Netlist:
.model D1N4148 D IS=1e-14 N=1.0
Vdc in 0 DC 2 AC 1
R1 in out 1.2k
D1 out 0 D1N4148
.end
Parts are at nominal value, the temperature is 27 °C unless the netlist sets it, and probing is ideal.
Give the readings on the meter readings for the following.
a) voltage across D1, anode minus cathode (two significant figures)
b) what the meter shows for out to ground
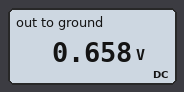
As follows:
660 mV
0.658 V
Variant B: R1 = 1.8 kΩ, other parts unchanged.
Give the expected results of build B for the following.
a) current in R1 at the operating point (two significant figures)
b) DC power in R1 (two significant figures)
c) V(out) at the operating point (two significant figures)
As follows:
750 µA
1.0 mW
650 mV
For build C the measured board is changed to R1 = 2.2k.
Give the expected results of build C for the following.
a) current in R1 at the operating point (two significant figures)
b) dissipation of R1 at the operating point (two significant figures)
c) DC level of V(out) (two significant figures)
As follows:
620 µA
840 µW
640 mV
